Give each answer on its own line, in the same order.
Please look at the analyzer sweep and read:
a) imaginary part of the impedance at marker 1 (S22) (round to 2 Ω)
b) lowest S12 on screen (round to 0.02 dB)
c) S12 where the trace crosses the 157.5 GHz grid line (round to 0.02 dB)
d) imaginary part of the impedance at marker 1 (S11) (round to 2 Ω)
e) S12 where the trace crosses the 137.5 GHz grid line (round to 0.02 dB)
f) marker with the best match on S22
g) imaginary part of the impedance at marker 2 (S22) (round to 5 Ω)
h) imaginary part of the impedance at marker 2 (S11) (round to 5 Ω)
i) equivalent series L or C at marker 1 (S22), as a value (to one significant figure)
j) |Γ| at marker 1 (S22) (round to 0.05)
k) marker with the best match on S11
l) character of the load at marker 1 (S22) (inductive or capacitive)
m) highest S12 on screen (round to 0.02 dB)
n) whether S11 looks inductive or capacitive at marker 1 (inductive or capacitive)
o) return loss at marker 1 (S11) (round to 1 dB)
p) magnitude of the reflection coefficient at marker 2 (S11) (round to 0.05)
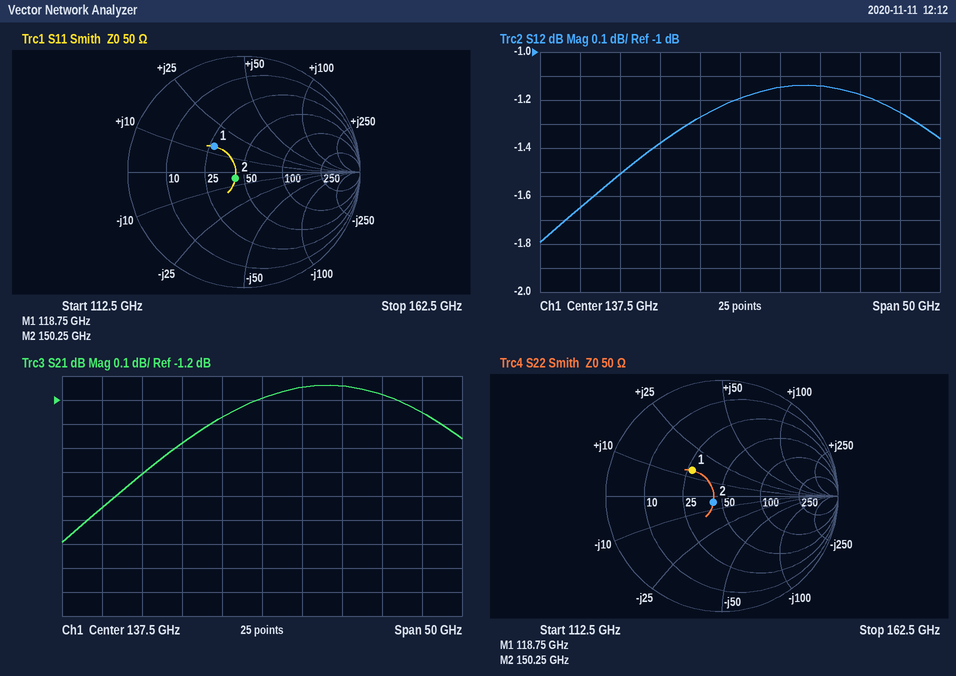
+14 Ω
-1.80 dB
-1.26 dB
+14 Ω
-1.20 dB
marker 2
-5 Ω
-5 Ω
20 pH
0.35
marker 2
inductive
-1.14 dB
inductive
9 dB
0.10
